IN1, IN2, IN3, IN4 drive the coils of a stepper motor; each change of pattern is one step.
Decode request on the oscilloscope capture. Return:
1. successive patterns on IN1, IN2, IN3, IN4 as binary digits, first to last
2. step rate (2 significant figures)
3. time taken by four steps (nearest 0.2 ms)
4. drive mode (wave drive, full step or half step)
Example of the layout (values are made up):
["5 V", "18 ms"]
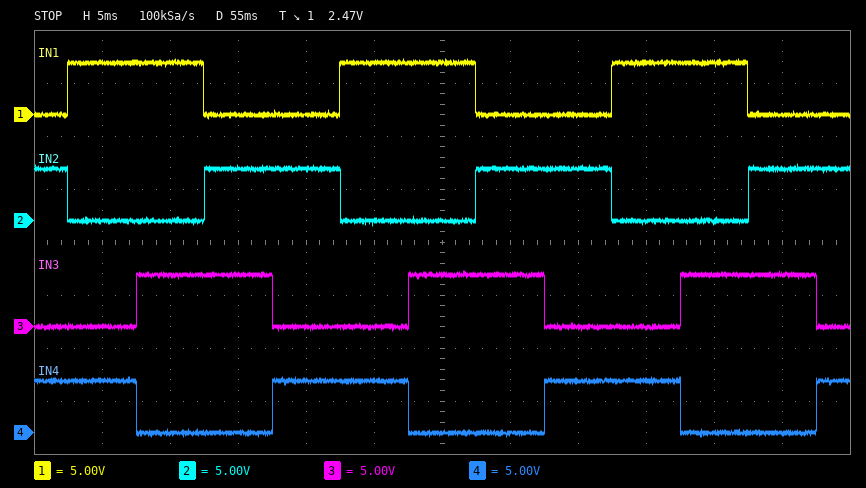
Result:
["0101 1001 1010 0110 0101 1001 1010 0110 0101 1001 1010 0110 0101", "200 steps/s", "20.0 ms", "full step"]
